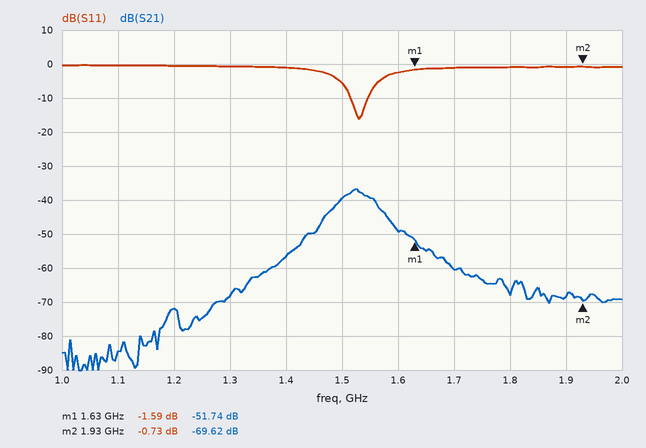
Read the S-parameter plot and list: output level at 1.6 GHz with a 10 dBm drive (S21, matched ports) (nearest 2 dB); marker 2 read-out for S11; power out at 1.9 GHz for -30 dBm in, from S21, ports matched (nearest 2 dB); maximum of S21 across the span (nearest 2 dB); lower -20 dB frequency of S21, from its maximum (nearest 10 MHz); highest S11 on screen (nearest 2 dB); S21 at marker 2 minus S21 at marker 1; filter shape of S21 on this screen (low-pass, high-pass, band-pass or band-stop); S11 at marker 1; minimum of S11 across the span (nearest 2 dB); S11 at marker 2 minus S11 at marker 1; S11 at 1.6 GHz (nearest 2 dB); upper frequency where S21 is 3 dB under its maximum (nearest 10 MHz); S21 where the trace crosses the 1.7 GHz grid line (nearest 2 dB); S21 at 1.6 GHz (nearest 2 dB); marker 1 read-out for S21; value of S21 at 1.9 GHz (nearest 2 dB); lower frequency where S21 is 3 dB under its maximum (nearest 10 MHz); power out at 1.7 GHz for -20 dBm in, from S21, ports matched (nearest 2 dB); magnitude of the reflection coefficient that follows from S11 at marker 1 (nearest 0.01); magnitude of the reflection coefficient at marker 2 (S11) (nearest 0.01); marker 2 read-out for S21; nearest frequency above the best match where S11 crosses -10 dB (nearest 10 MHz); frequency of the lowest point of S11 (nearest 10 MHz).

-40 dBm
-0.73 dB
-98 dBm
-36 dB
1.40 GHz
0 dB
-17.88 dB
band-pass
-1.59 dB
-16 dB
0.86 dB
-2 dB
1.56 GHz
-60 dB
-50 dB
-51.74 dB
-68 dB
1.50 GHz
-80 dBm
0.83
0.92
-69.62 dB
1.55 GHz
1.53 GHz
